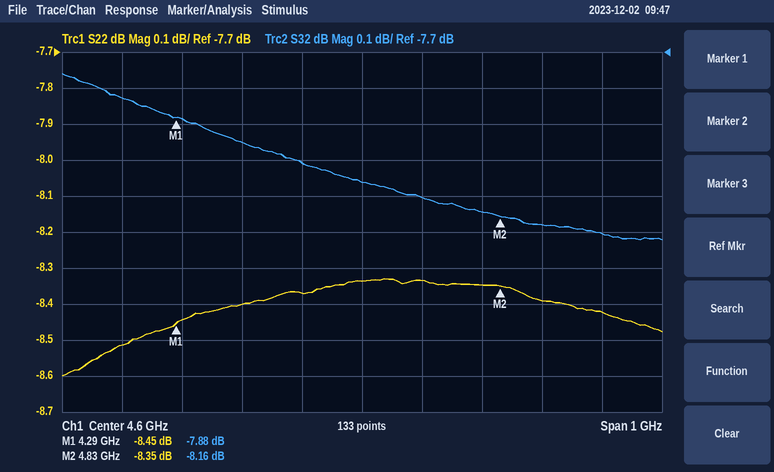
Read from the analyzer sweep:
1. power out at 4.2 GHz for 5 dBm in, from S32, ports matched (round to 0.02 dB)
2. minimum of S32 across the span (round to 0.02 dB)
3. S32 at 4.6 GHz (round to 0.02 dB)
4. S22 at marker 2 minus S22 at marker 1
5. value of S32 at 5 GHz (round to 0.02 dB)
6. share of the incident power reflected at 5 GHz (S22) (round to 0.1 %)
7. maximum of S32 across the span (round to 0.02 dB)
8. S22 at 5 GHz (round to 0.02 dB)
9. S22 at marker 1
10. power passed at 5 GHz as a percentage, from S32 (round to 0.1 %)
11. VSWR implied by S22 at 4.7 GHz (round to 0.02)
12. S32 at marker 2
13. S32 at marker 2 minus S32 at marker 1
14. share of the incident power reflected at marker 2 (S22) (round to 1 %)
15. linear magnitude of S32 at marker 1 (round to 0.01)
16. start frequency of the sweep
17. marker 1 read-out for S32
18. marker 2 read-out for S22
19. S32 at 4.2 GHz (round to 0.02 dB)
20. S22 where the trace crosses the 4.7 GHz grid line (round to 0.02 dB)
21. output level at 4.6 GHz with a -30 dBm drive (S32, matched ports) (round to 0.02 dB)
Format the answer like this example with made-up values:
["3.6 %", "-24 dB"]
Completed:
["-2.82 dBm", "-8.22 dB", "-8.06 dB", "0.10 dB", "-8.20 dB", "14.4 %", "-7.76 dB", "-8.42 dB", "-8.45 dB", "15.1 %", "2.24", "-8.16 dB", "-0.28 dB", "15 %", "0.40", "4.1 GHz", "-7.88 dB", "-8.35 dB", "-7.82 dB", "-8.34 dB", "-38.06 dBm"]
